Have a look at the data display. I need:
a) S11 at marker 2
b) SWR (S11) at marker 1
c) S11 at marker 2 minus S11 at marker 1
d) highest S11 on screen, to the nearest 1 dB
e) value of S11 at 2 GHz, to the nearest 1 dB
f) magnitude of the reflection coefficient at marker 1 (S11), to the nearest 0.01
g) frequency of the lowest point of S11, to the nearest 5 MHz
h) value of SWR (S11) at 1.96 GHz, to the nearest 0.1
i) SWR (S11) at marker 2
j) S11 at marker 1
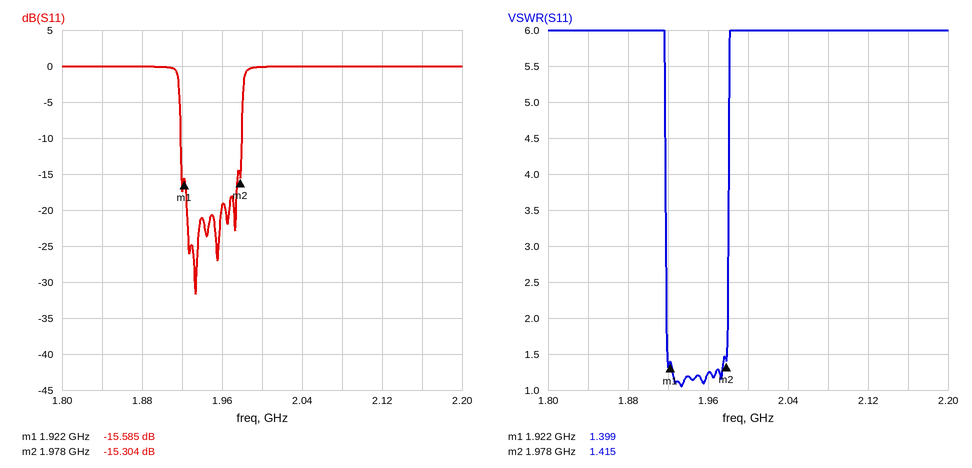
-15.304 dB
1.399
0.281 dB
0 dB
0 dB
0.17
1.935 GHz
1.2
1.415
-15.585 dB
